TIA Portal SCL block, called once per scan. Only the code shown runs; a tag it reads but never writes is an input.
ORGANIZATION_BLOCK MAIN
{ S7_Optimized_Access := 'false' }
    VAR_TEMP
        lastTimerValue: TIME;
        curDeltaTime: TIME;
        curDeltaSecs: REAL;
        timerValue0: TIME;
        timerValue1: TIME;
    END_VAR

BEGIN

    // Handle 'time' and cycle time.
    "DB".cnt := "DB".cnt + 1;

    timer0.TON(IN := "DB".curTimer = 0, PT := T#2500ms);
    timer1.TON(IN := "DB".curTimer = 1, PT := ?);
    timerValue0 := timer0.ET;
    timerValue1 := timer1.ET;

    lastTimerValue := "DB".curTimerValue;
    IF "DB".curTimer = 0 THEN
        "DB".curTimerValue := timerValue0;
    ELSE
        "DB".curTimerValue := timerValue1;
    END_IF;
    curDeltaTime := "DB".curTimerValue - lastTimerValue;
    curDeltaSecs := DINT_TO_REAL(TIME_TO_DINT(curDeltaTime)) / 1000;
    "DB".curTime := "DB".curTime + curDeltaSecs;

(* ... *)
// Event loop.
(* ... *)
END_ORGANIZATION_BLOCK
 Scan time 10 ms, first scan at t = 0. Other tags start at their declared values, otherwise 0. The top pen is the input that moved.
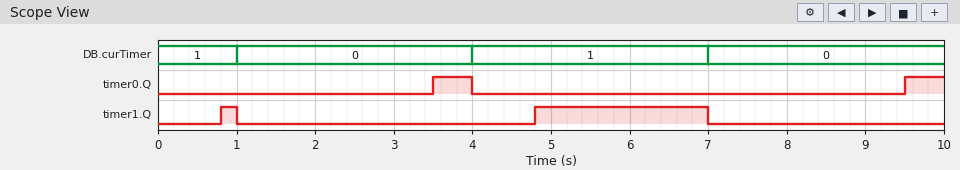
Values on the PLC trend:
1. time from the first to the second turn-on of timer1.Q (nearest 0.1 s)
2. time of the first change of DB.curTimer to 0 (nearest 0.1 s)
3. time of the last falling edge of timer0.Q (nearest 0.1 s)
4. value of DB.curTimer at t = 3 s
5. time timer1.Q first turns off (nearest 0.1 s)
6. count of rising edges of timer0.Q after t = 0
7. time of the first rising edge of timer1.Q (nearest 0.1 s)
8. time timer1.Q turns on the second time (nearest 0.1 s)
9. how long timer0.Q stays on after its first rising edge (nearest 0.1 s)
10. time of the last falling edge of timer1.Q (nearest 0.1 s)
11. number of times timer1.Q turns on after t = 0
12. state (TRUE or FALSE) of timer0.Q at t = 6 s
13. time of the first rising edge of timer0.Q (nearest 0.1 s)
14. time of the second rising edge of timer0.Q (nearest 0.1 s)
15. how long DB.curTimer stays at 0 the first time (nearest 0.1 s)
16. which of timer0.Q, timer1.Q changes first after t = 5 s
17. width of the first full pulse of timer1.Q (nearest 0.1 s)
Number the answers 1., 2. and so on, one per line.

1. 4.0 s
2. 1.0 s
3. 4.0 s
4. 0
5. 1.0 s
6. 2
7. 0.8 s
8. 4.8 s
9. 0.5 s
10. 7.0 s
11. 2
12. FALSE
13. 3.5 s
14. 9.5 s
15. 3.0 s
16. timer1.Q
17. 0.2 s
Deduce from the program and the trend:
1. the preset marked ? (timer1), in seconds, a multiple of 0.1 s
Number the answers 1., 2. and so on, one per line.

1. 0.8 s
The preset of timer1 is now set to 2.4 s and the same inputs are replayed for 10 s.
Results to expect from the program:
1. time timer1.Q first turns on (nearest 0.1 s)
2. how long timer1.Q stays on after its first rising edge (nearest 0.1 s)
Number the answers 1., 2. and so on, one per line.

1. 6.4 s
2. 0.6 s
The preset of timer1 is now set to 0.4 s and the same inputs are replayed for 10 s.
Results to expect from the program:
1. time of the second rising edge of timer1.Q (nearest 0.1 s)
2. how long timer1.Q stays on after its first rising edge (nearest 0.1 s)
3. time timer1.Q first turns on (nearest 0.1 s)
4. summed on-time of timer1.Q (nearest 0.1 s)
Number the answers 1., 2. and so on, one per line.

1. 4.4 s
2. 0.6 s
3. 0.4 s
4. 3.2 s
